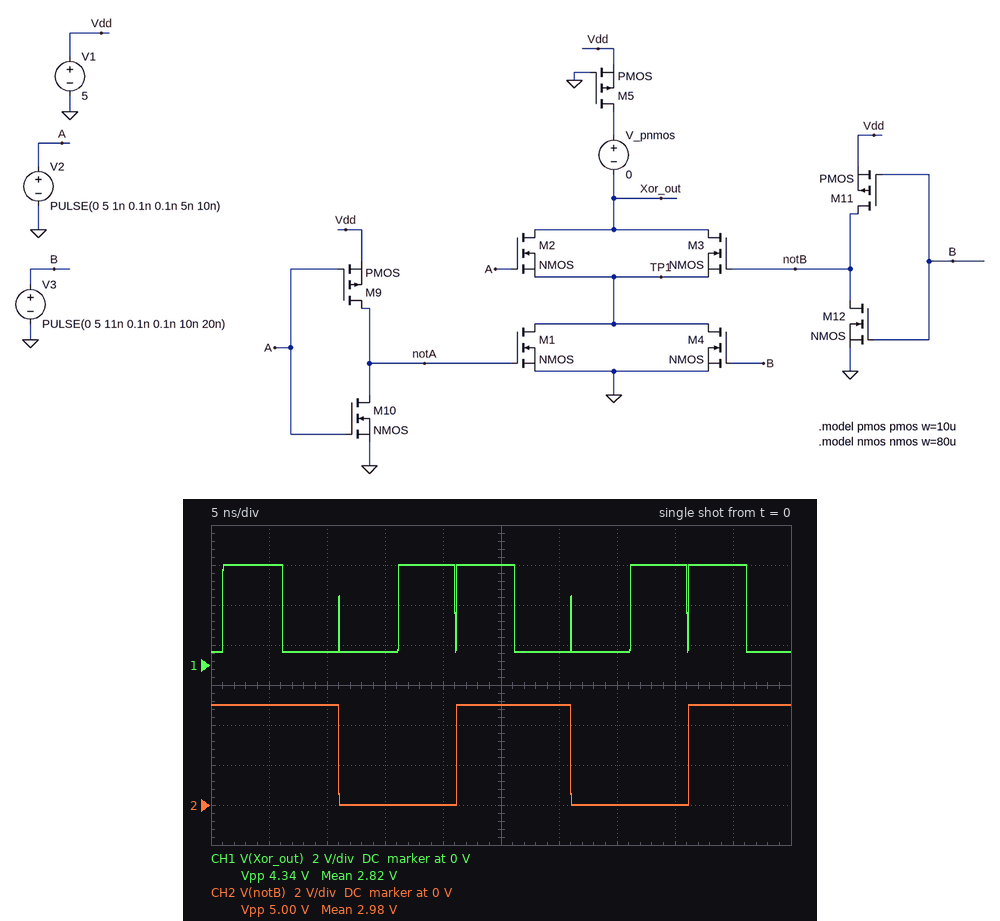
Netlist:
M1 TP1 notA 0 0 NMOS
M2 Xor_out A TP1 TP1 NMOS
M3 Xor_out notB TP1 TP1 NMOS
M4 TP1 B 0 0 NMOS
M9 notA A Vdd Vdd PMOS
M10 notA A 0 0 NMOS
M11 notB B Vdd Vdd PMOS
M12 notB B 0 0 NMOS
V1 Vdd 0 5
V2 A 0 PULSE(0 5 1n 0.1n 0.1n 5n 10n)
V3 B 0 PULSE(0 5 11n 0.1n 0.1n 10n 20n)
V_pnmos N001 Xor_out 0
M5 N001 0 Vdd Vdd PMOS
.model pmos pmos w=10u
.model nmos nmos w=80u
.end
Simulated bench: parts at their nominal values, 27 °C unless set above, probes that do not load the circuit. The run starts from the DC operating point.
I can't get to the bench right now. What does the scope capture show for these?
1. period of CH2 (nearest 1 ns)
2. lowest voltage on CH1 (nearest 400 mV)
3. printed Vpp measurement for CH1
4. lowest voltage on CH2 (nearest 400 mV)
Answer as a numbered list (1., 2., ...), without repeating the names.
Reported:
1. 20 ns
2. 800 mV
3. 4.34 V
4. 0 V
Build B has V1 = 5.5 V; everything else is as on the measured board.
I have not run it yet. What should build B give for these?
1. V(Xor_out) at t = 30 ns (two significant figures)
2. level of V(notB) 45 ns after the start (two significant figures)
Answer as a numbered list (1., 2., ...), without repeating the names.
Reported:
1. 720 mV
2. 5.5 V
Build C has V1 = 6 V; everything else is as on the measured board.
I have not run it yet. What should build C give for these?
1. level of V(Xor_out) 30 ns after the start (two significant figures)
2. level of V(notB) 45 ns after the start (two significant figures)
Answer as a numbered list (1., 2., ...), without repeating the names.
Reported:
1. 790 mV
2. 6.0 V
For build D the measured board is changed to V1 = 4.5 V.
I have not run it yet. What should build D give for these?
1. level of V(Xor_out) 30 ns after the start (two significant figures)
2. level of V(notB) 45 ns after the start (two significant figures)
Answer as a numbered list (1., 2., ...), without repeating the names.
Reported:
1. 590 mV
2. 4.5 V
